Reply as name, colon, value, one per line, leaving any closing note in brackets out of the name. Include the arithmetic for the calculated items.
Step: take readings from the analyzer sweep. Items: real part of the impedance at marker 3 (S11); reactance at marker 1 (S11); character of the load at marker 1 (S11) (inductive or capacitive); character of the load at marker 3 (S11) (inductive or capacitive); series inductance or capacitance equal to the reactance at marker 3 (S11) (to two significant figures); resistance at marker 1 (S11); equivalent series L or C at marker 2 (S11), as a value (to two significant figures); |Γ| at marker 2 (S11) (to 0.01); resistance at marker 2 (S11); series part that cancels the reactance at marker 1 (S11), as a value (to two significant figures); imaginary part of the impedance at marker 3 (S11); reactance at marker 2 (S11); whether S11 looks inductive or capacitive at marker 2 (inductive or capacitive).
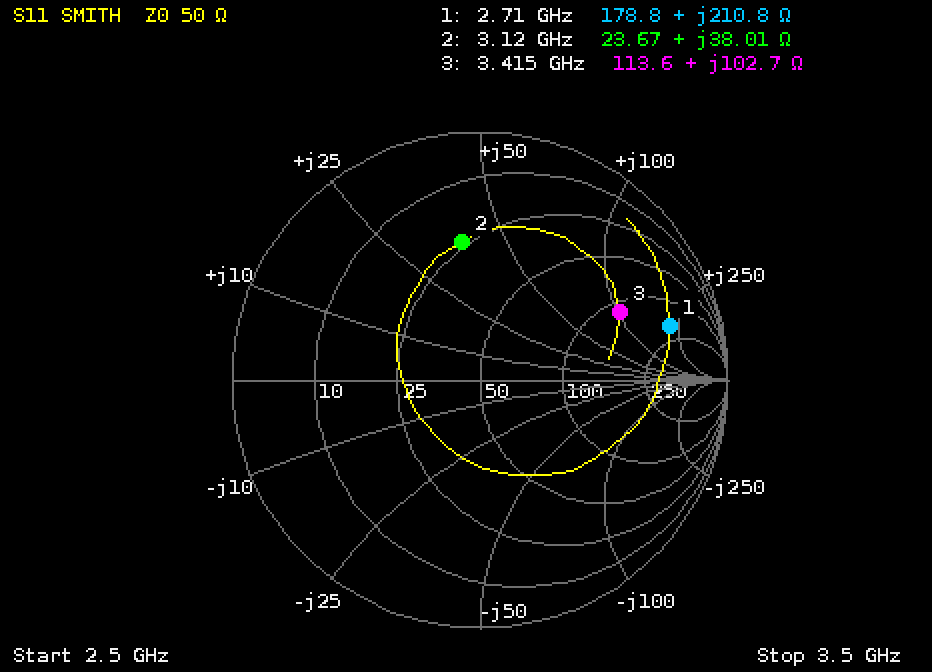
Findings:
real part of the impedance at marker 3: 113.6 Ω
reactance at marker 1: +210.8 Ω
character of the load at marker 1 (S11): inductive
character of the load at marker 3 (S11): inductive
series inductance or capacitance equal to the reactance at marker 3 (S11): L = 102.7 Ω/(2π × 3.415 GHz) ≈ 4.8 nH
resistance at marker 1: 178.8 Ω
equivalent series L or C at marker 2 (S11), as a value: L = 38.01 Ω/(2π × 3.12 GHz) ≈ 1.9 nH
|Γ| at marker 2 (S11): 0.56
resistance at marker 2: 23.67 Ω
series part that cancels the reactance at marker 1 (S11), as a value: C = 1/(2π × 2.71 GHz × 210.8 Ω) ≈ 279 fF, so 280 fF to two significant figures
imaginary part of the impedance at marker 3: +102.7 Ω
reactance at marker 2: +38.01 Ω
whether S11 looks inductive or capacitive at marker 2: inductive
